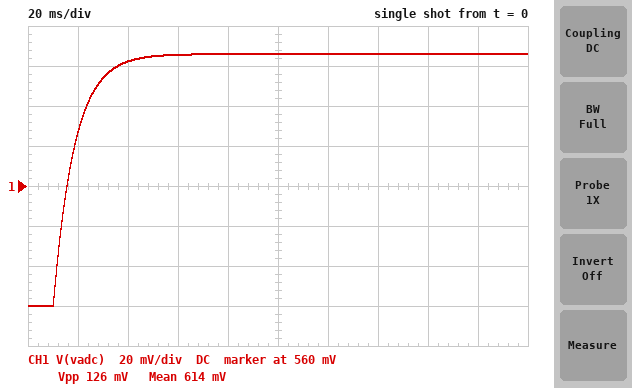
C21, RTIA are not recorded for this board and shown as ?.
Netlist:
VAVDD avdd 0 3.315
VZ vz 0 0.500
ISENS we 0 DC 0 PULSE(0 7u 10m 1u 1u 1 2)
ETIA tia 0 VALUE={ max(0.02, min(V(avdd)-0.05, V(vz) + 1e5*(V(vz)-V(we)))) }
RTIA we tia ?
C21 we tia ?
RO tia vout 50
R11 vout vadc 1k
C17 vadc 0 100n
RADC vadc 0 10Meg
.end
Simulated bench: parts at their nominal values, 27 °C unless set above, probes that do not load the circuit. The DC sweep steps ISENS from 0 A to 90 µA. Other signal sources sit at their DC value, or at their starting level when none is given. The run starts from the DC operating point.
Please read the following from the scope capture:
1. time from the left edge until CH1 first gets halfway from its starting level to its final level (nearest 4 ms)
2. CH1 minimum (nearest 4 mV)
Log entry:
16 ms
500 mV
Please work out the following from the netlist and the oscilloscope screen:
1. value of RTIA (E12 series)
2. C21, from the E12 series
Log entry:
18 kΩ
470 nF
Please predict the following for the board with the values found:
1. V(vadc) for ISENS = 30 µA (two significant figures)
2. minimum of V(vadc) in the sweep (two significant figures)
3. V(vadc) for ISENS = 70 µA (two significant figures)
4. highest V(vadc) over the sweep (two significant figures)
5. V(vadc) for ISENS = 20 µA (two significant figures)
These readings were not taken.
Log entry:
1.0 V
500 mV
1.8 V
2.1 V
860 mV
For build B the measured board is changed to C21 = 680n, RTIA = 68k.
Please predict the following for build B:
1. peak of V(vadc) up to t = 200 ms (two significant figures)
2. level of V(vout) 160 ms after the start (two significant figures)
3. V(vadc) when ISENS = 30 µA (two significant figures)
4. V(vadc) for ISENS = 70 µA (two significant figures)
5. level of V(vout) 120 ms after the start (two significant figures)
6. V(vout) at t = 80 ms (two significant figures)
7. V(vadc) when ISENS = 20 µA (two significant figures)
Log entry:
970 mV
960 mV
2.5 V
3.3 V
930 mV
870 mV
1.9 V
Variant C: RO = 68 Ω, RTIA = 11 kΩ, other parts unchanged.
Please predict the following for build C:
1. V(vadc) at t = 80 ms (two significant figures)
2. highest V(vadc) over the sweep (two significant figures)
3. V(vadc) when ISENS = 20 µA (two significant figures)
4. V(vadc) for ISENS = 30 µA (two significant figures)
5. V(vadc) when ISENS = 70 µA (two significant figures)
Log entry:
580 mV
1.5 V
720 mV
830 mV
1.3 V
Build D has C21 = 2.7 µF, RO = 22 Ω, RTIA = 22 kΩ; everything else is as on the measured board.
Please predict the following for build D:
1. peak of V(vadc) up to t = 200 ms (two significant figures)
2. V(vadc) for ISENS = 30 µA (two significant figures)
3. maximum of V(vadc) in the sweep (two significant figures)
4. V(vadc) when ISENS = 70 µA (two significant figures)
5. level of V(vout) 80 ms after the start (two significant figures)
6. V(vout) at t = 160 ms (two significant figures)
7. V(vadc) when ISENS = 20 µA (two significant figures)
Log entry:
650 mV
1.2 V
2.5 V
2.0 V
610 mV
640 mV
940 mV
